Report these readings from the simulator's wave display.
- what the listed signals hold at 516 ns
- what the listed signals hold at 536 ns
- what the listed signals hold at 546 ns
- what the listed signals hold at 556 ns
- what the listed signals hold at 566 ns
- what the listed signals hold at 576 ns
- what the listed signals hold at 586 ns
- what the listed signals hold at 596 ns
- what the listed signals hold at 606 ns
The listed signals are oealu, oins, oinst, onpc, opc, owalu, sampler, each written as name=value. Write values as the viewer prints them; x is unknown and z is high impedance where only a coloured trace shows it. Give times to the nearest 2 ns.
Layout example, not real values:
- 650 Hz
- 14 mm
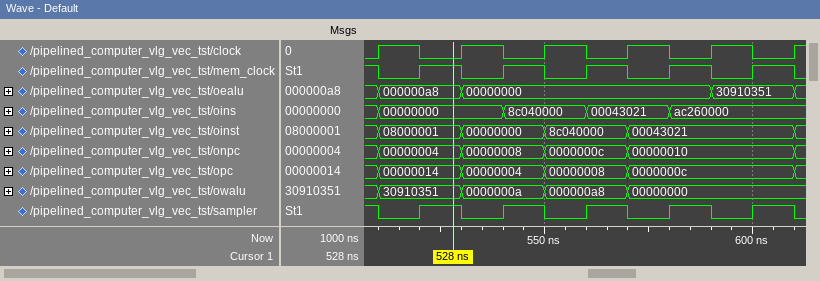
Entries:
- oealu=000000a8, oins=00000000, oinst=08000001, onpc=00000004, opc=00000014, owalu=30910351, sampler=0
- oealu=00000000, oins=00000000, oinst=00000000, onpc=00000008, opc=00000004, owalu=0000000a, sampler=0
- oealu=00000000, oins=8c040000, oinst=00000000, onpc=00000008, opc=00000004, owalu=0000000a, sampler=1
- oealu=00000000, oins=8c040000, oinst=8c040000, onpc=0000000c, opc=00000008, owalu=000000a8, sampler=0
- oealu=00000000, oins=00043021, oinst=8c040000, onpc=0000000c, opc=00000008, owalu=000000a8, sampler=1
- oealu=00000000, oins=00043021, oinst=00043021, onpc=00000010, opc=0000000c, owalu=00000000, sampler=0
- oealu=00000000, oins=ac260000, oinst=00043021, onpc=00000010, opc=0000000c, owalu=00000000, sampler=1
- oealu=30910351, oins=ac260000, oinst=00043021, onpc=00000010, opc=0000000c, owalu=00000000, sampler=0
- oealu=30910351, oins=ac260000, oinst=00043021, onpc=00000010, opc=0000000c, owalu=00000000, sampler=1
